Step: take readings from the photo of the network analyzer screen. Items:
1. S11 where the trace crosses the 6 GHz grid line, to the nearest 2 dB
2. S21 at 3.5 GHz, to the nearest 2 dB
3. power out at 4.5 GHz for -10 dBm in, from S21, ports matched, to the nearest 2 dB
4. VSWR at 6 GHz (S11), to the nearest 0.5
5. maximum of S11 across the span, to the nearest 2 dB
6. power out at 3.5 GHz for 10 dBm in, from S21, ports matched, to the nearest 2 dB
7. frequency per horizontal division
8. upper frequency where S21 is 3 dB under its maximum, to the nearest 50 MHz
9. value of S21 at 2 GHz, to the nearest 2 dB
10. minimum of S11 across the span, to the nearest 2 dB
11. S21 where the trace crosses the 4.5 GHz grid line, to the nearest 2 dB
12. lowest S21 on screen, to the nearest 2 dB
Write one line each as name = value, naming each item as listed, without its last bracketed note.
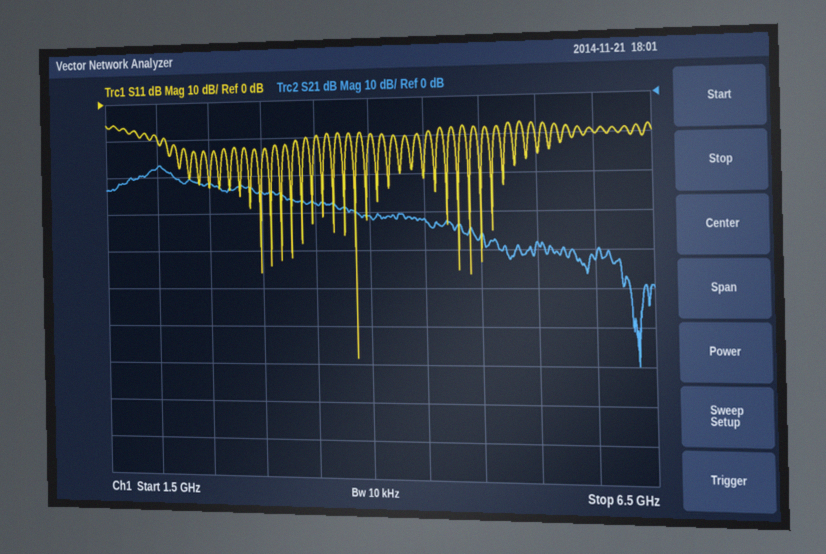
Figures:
S11 where the trace crosses the 6 GHz grid line, to the nearest 2 dB = -10 dB
S21 at 3.5 GHz, to the nearest 2 dB = -28 dB
power out at 4.5 GHz for -10 dBm in, from S21, ports matched, to the nearest 2 dB = -42 dBm
VSWR at 6 GHz (S11), to the nearest 0.5 = 2.0
maximum of S11 across the span, to the nearest 2 dB = -6 dB
power out at 3.5 GHz for 10 dBm in, from S21, ports matched, to the nearest 2 dB = -18 dBm
frequency per horizontal division = 500 MHz
upper frequency where S21 is 3 dB under its maximum, to the nearest 50 MHz = 2.15 GHz
value of S21 at 2 GHz, to the nearest 2 dB = -18 dB
minimum of S11 across the span, to the nearest 2 dB = -68 dB
S21 where the trace crosses the 4.5 GHz grid line, to the nearest 2 dB = -32 dB
lowest S21 on screen, to the nearest 2 dB = -70 dB
